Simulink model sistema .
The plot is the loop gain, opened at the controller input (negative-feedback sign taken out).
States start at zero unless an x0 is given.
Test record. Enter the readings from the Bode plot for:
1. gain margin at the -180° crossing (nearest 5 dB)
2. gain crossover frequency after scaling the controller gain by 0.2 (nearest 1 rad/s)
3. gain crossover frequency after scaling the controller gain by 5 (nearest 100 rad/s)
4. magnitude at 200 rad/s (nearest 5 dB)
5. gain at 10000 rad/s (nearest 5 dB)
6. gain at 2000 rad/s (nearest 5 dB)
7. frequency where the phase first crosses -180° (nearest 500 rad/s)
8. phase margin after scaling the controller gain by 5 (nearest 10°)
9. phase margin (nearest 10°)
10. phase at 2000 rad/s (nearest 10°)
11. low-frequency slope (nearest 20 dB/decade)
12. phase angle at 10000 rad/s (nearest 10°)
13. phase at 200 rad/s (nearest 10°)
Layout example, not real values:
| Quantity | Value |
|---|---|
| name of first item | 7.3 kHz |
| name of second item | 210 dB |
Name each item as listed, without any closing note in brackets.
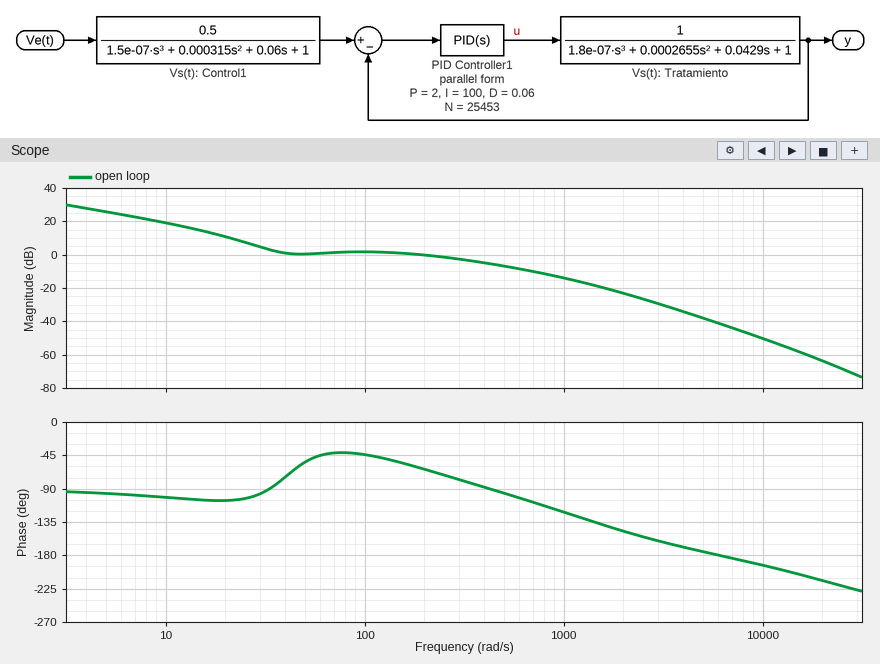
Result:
| Quantity | Value |
|---|---|
| gain margin at the -180° crossing | 40 dB |
| gain crossover frequency after scaling the controller gain by 0.2 | 16 rad/s |
| gain crossover frequency after scaling the controller gain by 5 | 1000 rad/s |
| magnitude at 200 rad/s | 0 dB |
| gain at 10000 rad/s | -50 dB |
| gain at 2000 rad/s | -25 dB |
| frequency where the phase first crosses -180° | 6000 rad/s |
| phase margin after scaling the controller gain by 5 | 60° |
| phase margin | 120° |
| phase at 2000 rad/s | -150° |
| low-frequency slope | -20 dB/decade |
| phase angle at 10000 rad/s | -190° |
| phase at 200 rad/s | -60° |
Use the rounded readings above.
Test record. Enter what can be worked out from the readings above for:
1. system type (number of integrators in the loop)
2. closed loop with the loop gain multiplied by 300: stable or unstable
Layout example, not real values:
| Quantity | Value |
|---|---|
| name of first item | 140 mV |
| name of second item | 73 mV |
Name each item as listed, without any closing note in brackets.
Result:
| Quantity | Value |
|---|---|
| system type | 1 |
| closed loop with the loop gain multiplied by 300: stable or unstable | unstable |
